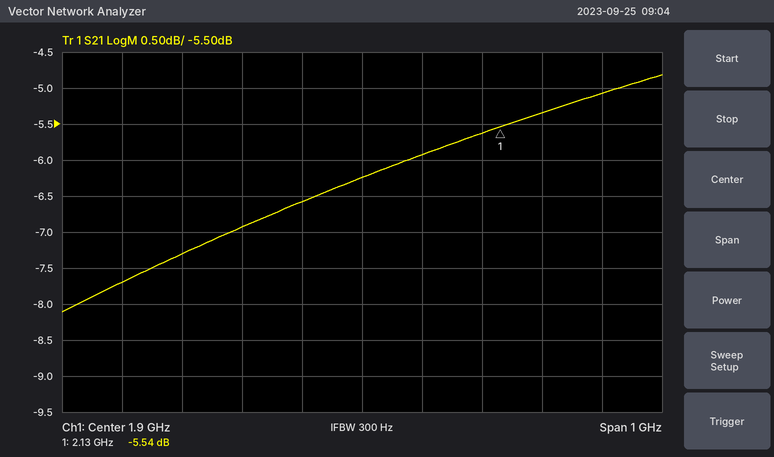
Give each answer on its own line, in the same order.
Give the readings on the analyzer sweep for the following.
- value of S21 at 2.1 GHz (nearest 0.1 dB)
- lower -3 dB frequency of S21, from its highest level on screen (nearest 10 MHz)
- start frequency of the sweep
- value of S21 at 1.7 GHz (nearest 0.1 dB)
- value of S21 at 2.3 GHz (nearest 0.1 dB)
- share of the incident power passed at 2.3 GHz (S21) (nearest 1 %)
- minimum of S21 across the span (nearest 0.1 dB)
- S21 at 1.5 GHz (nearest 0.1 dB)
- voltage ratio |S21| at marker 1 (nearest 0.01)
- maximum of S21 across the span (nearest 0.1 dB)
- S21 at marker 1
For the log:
-5.6 dB
1.47 GHz
1.4 GHz
-6.9 dB
-5.1 dB
31 %
-8.1 dB
-7.7 dB
0.53
-4.8 dB
-5.54 dB
